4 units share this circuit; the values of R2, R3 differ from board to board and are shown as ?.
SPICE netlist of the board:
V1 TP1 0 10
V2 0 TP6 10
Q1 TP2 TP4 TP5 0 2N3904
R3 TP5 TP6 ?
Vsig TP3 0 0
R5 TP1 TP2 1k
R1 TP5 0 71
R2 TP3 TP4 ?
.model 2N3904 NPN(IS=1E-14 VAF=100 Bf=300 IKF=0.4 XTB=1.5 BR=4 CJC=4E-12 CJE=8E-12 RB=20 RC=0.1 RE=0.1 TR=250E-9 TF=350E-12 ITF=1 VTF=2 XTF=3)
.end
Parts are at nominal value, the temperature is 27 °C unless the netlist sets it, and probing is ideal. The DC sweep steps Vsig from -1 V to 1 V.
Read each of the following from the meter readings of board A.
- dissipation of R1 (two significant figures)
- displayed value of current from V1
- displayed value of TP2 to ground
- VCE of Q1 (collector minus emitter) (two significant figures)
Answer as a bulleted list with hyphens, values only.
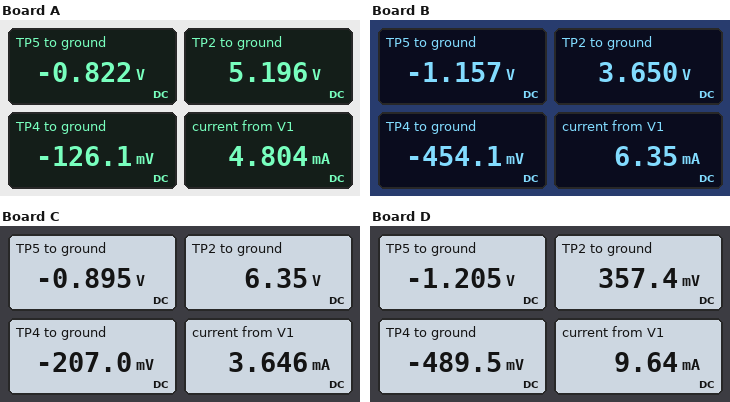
- 9.5 mW
- 4.804 mA
- 5.196 V
- 6.0 V
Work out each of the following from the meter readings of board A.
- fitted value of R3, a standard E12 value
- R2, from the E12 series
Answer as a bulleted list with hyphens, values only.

- 560 Ω
- 8.2 kΩ
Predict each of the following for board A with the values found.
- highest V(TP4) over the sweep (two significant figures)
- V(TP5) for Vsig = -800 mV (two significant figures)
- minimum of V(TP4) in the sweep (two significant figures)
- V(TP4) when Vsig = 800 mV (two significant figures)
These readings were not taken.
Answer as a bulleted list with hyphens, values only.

- 250 mV
- -1.1 V
- -1.0 V
- 250 mV
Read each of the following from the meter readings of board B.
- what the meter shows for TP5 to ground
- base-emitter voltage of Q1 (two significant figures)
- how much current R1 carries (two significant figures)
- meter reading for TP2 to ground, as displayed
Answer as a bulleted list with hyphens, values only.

- -1.157 V
- 700 mV
- 16 mA
- 3.650 V
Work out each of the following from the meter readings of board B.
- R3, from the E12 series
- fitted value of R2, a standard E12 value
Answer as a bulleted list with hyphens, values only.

- 390 Ω
- 22 kΩ
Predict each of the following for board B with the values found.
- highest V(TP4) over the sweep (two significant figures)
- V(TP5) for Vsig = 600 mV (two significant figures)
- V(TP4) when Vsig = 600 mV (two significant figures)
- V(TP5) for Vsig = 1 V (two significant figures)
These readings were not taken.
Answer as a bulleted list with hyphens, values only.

- -170 mV
- -910 mV
- -190 mV
- -890 mV
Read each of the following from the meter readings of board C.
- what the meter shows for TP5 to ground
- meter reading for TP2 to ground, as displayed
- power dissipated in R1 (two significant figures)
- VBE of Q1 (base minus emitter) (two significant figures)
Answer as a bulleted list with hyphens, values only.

- -0.895 V
- 6.35 V
- 11 mW
- 690 mV
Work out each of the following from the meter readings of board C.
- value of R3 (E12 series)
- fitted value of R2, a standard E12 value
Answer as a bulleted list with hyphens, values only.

- 560 Ω
- 18 kΩ
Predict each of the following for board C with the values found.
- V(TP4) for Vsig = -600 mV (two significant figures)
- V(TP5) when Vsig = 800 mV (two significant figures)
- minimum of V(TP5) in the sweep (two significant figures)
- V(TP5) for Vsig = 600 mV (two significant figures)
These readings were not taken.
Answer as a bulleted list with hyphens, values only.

- -600 mV
- -510 mV
- -1.1 V
- -610 mV
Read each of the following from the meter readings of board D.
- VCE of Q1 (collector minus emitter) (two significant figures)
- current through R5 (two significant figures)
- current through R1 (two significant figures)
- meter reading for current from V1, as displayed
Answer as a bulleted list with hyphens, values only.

- 1.6 V
- 9.6 mA
- 17 mA
- 9.64 mA
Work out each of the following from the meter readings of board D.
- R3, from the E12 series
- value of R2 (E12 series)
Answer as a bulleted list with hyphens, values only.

- 330 Ω
- 15 kΩ
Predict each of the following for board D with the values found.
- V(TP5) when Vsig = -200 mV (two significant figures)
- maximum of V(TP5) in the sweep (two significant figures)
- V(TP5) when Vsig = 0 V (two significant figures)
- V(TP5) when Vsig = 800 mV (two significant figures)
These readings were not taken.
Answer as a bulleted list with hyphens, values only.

- -1.3 V
- -1.1 V
- -1.2 V
- -1.1 V
